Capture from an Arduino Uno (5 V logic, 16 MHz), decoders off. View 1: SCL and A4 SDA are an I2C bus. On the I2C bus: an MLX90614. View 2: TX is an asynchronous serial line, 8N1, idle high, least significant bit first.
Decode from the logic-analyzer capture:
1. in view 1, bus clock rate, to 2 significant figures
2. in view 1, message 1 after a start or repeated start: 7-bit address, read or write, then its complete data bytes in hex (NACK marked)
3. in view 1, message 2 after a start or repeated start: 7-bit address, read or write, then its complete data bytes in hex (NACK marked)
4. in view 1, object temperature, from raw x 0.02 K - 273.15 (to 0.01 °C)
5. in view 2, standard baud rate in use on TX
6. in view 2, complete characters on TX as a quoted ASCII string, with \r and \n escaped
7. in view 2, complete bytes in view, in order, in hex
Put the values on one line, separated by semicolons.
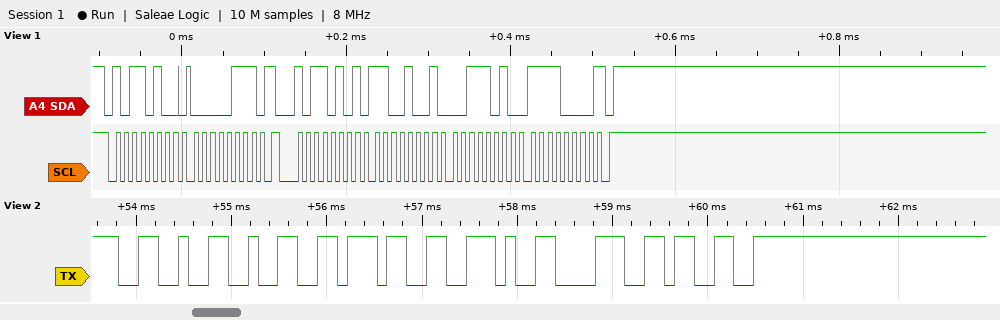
100 kHz; 0x5A write: 07; 0x5A read: C9 3A F0 NACK; 27.83 °C; 9600 baud; "&27.83"; 26 32 37 2E 38 33
